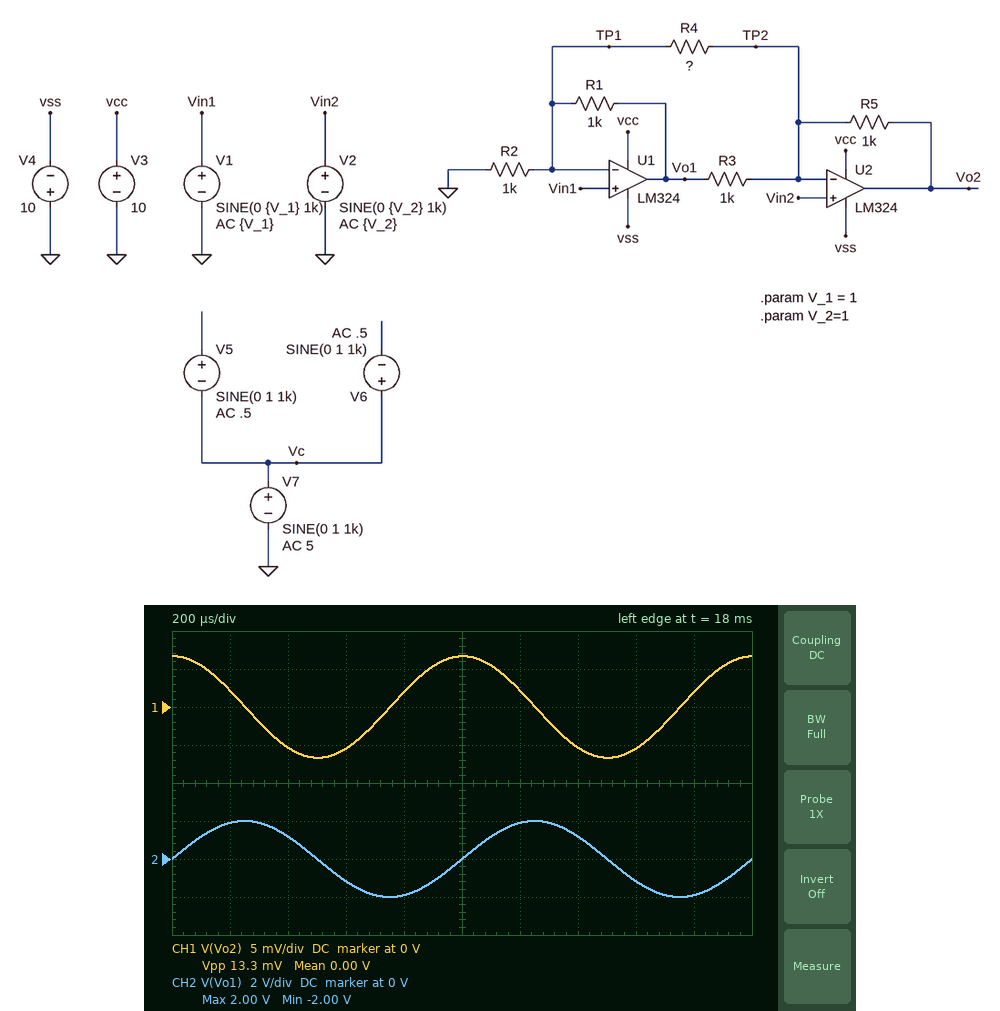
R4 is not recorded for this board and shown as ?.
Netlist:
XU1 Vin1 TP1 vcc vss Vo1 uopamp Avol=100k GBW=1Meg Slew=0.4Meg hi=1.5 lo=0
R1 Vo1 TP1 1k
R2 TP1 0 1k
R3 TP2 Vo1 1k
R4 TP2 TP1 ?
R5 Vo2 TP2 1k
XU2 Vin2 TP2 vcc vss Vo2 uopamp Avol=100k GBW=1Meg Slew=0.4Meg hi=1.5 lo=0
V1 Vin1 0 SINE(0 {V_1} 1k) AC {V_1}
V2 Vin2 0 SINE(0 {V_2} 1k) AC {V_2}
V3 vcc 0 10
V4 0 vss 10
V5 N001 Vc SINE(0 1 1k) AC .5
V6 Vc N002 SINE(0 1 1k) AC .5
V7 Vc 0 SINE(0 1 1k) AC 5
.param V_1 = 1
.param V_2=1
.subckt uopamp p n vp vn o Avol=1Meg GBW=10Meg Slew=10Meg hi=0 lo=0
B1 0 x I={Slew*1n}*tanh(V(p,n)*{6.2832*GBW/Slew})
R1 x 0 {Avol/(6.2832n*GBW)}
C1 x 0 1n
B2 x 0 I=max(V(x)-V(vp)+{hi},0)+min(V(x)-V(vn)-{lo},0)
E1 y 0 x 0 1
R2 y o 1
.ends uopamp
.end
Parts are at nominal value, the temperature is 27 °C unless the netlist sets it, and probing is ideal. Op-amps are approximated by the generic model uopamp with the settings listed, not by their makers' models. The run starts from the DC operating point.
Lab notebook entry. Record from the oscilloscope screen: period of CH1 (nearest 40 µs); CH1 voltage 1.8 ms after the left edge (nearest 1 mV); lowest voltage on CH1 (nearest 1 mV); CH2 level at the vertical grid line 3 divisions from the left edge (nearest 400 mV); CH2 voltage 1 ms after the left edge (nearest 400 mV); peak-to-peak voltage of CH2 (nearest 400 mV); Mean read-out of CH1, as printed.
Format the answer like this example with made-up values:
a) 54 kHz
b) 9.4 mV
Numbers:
a) 1.00 ms
b) 2 mV
c) -7 mV
d) -1.2 V
e) 0 V
f) 4.0 V
g) 0.00 V
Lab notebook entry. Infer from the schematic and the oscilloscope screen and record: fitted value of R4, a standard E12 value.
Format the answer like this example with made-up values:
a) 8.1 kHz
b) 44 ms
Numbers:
a) 1.5 kΩ
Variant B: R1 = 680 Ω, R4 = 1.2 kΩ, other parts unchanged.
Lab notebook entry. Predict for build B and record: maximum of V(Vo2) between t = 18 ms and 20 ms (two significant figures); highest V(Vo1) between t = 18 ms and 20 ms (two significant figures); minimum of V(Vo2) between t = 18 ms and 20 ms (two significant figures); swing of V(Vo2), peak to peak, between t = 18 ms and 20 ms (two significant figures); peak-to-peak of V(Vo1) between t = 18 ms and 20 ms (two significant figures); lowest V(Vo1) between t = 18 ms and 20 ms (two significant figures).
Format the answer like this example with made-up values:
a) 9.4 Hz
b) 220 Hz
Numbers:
a) 320 mV
b) 1.7 V
c) -320 mV
d) 640 mV
e) 3.4 V
f) -1.7 V
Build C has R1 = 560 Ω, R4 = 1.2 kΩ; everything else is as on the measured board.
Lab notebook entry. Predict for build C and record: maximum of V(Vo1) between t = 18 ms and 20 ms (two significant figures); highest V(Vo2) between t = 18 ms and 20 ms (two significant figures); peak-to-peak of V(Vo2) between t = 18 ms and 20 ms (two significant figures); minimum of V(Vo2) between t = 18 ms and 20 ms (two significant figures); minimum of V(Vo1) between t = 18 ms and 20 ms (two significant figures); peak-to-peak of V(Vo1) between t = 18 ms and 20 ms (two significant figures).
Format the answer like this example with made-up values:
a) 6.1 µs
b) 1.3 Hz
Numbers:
a) 1.6 V
b) 440 mV
c) 880 mV
d) -440 mV
e) -1.6 V
f) 3.1 V
